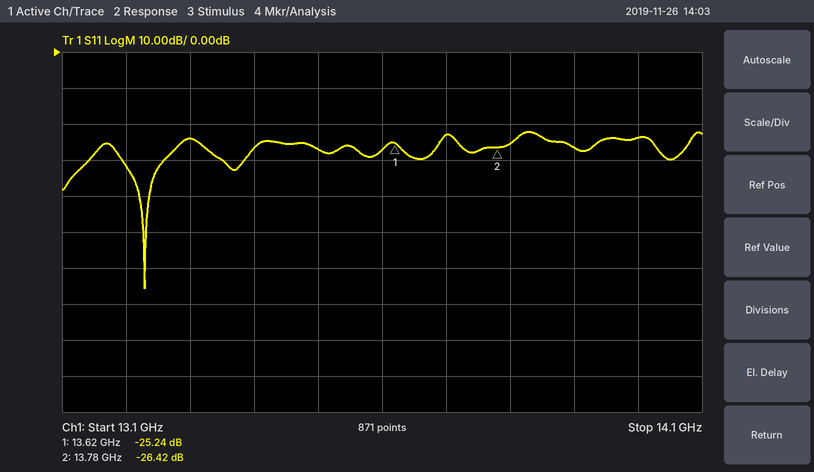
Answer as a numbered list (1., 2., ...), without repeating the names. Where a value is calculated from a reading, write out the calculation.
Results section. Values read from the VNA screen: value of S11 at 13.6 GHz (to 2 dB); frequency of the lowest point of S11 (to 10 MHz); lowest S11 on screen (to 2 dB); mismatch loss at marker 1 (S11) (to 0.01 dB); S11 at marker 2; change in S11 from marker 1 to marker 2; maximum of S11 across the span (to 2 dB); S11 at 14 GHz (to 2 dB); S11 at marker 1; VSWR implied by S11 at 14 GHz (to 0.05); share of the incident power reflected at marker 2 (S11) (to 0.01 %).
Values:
1. -28 dB
2. 13.23 GHz
3. -66 dB
4. −10 log10(1 − 10^(-25.24/10)) ≈ 0.01 dB
5. -26.42 dB
6. -26.42 − (-25.24) = -1.18 dB
7. -22 dB
8. -24 dB
9. -25.24 dB
10. |Γ| = 10^(-24/20) = 0.0631; VSWR = (1 + 0.0631)/(1 − 0.0631) ≈ 1.13, so 1.15 to the nearest 0.05
11. 10^(-26.42/10) ≈ 0.23 %
